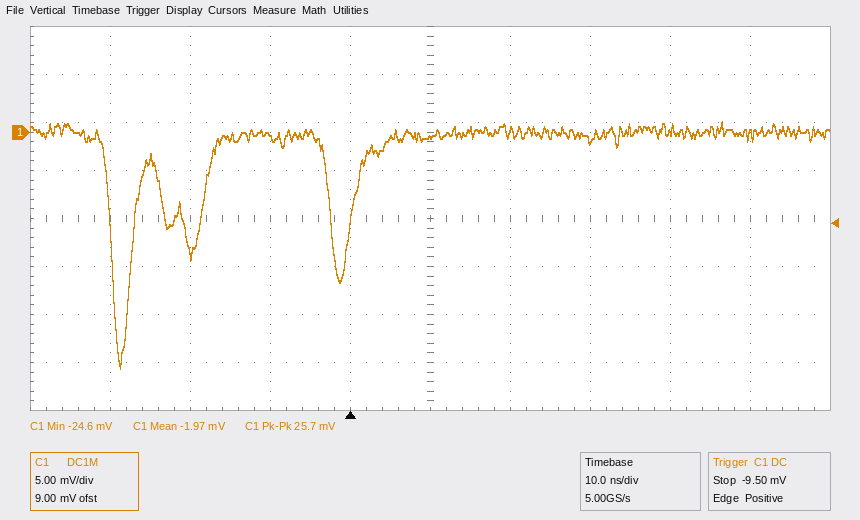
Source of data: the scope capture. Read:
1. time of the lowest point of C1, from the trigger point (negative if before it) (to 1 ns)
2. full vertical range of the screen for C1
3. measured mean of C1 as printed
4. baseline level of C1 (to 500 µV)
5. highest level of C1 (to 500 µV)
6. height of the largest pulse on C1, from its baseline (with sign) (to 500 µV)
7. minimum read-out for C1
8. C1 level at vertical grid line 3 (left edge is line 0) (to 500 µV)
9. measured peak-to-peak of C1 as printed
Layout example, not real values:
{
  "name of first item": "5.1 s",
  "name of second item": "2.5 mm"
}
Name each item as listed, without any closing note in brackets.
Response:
{
  "time of the lowest point of C1, from the trigger point (negative if before it)": "-29 ns",
  "full vertical range of the screen for C1": "40 mV",
  "measured mean of C1 as printed": "-1.97 mV",
  "baseline level of C1": "0.0 mV",
  "highest level of C1": "1.0 mV",
  "height of the largest pulse on C1, from its baseline (with sign)": "-24.5 mV",
  "minimum read-out for C1": "-24.6 mV",
  "C1 level at vertical grid line 3 (left edge is line 0)": "-500 µV",
  "measured peak-to-peak of C1 as printed": "25.7 mV"
}
